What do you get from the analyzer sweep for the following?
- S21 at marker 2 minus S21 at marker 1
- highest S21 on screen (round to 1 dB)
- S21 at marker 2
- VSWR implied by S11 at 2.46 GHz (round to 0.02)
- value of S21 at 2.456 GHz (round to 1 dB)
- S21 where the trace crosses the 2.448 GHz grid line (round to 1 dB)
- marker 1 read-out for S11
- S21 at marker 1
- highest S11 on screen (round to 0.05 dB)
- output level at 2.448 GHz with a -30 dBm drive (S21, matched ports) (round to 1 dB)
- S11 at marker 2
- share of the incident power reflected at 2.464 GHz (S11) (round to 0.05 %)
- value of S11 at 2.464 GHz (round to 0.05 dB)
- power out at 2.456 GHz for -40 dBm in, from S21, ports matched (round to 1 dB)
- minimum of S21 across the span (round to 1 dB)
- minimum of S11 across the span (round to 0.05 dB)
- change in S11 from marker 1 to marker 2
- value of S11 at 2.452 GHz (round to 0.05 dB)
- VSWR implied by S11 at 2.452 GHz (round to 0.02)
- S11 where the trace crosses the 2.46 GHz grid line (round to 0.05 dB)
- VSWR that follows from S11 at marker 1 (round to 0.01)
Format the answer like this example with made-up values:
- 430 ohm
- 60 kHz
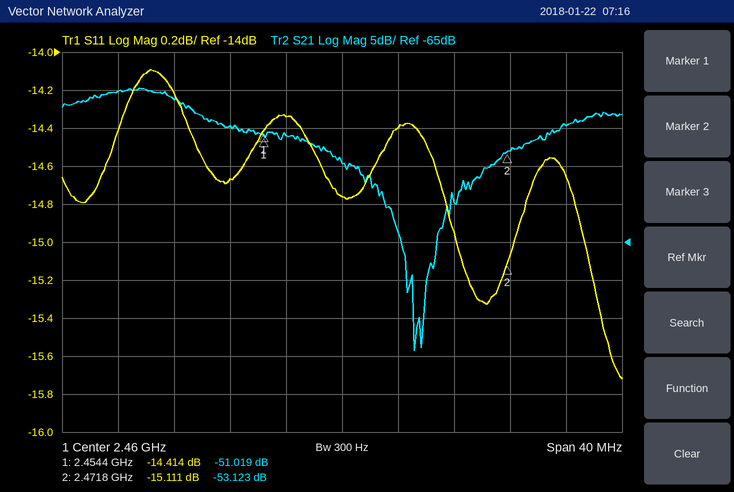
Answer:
- -2.104 dB
- -45 dB
- -53.123 dB
- 1.44
- -51 dB
- -46 dB
- -14.414 dB
- -51.019 dB
- -14.10 dB
- -76 dBm
- -15.111 dB
- 3.65 %
- -14.40 dB
- -91 dBm
- -79 dB
- -15.70 dB
- -0.697 dB
- -14.65 dB
- 1.46
- -14.75 dB
- 1.47
